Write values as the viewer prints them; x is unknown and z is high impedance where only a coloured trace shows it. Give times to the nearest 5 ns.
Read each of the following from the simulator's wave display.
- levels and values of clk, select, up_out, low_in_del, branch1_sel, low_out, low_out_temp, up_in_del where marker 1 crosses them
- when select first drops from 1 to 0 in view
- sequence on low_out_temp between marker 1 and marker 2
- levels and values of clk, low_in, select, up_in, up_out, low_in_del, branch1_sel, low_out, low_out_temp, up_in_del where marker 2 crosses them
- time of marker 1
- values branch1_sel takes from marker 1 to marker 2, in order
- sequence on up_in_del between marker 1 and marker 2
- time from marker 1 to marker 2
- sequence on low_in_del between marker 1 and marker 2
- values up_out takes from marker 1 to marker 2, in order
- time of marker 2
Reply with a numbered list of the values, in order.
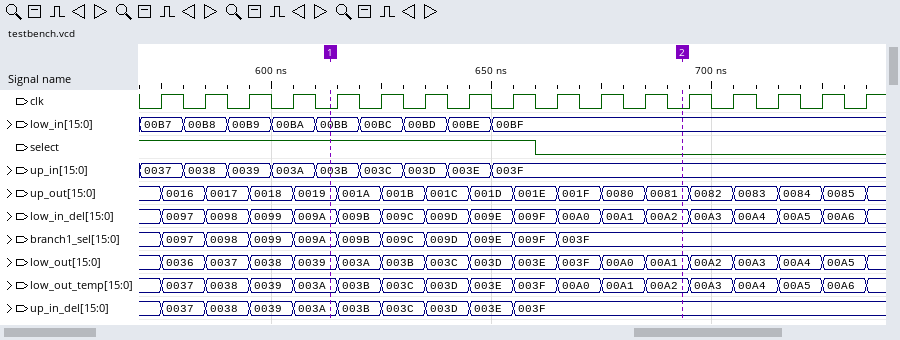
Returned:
1. clk=0, select=1, up_out=0019, low_in_del=009A, branch1_sel=009A, low_out=0039, low_out_temp=003A, up_in_del=003A
2. 660 ns
3. 003A, 003B, 003C, 003D, 003E, 003F, 00A0, 00A1, 00A2
4. clk=0, low_in=00BF, select=0, up_in=003F, up_out=0081, low_in_del=00A2, branch1_sel=003F, low_out=00A1, low_out_temp=00A2, up_in_del=003F
5. 615 ns
6. 009A, 009B, 009C, 009D, 009E, 009F, 003F
7. 003A, 003B, 003C, 003D, 003E, 003F
8. 80 ns
9. 009A, 009B, 009C, 009D, 009E, 009F, 00A0, 00A1, 00A2
10. 0019, 001A, 001B, 001C, 001D, 001E, 001F, 0080, 0081
11. 695 ns
